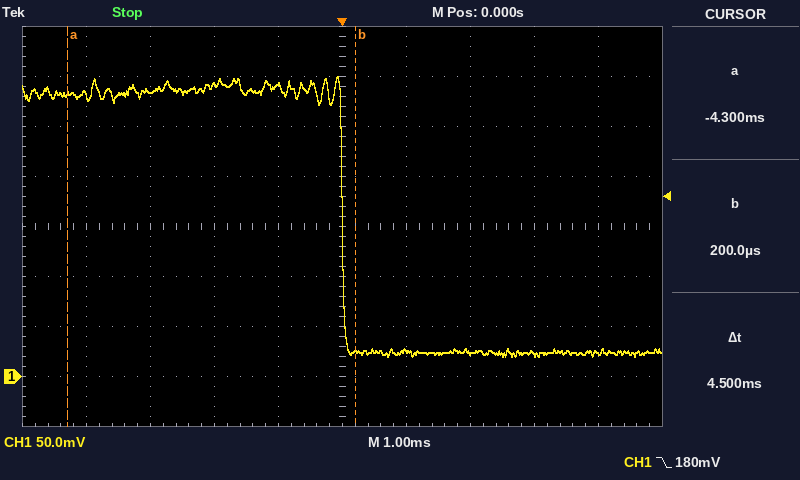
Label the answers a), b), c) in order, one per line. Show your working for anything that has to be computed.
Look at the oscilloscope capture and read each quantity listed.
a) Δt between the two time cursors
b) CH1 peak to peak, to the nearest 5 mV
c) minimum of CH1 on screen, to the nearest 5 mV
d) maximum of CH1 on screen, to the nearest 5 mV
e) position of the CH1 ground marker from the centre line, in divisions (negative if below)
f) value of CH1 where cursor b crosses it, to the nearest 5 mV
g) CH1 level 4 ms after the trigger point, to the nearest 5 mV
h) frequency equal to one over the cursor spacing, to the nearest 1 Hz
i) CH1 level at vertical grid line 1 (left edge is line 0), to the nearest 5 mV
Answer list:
a) 4.5 ms
b) 300 mV − (20 mV) = 280 mV
c) 20 mV
d) 300 mV
e) -3.0 div
f) 25 mV
g) 25 mV
h) 1 / 4.5 ms ≈ 222 Hz
i) 280 mV
